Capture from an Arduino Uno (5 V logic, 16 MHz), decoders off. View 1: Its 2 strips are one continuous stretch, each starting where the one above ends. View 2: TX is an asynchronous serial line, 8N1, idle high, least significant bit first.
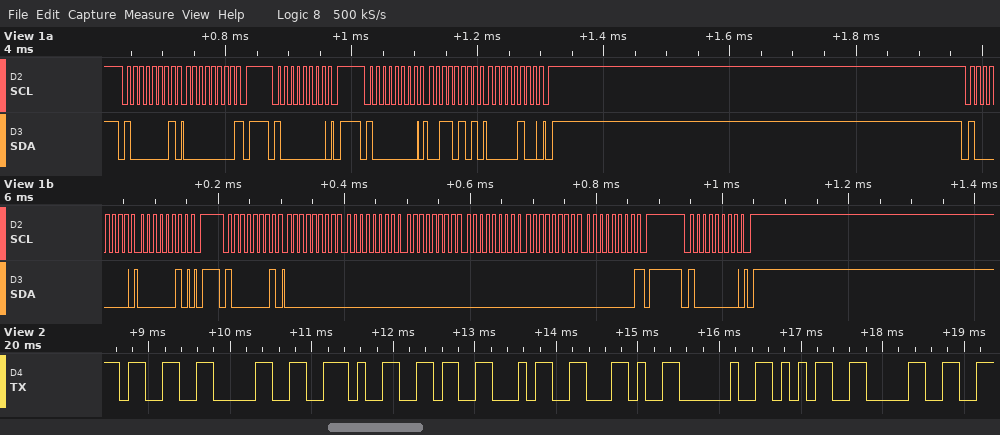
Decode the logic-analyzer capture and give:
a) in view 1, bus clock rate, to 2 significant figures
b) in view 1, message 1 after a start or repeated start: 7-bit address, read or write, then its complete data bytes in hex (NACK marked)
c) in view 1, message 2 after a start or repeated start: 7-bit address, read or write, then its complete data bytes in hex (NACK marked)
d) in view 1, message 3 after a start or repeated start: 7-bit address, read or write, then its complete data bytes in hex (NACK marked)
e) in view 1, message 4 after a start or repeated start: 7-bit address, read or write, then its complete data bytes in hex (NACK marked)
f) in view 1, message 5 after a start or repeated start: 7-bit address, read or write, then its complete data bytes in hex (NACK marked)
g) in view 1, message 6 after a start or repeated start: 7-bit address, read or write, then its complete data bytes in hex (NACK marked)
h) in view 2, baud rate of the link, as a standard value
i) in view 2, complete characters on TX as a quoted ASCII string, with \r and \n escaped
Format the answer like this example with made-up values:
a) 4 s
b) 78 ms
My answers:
a) 100 kHz
b) 0x40 read: 00 NACK
c) 0x40 write
d) 0x40 write: 35 04
e) 0x40 write: 02
f) 0x40 read: 00 00 00 00 00 00 NACK
g) 0x40 write
h) 9600 baud
i) "30.64, 50"
